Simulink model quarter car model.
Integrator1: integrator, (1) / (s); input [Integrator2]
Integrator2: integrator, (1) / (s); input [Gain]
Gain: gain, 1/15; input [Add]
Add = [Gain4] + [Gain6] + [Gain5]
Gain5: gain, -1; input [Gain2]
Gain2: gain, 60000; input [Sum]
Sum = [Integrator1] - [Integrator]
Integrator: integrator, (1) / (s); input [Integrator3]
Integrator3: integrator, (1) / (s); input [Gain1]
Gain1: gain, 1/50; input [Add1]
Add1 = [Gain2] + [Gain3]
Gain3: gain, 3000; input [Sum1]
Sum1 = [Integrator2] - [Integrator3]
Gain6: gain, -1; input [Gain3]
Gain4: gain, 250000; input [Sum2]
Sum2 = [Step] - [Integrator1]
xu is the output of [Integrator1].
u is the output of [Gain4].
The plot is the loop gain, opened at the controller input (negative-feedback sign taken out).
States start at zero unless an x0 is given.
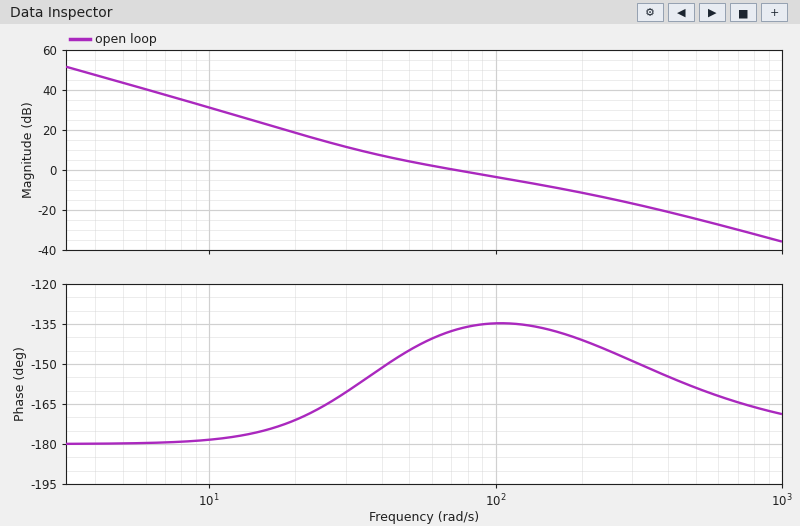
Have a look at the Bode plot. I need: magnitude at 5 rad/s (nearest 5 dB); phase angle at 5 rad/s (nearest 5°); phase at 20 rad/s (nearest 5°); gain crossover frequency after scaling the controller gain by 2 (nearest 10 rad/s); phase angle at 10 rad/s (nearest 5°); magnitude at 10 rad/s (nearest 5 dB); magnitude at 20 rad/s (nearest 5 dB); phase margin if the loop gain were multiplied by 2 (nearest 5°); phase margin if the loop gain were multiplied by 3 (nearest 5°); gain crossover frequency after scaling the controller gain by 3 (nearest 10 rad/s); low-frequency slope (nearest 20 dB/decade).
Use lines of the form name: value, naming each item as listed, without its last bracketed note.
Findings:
magnitude at 5 rad/s: 45 dB
phase angle at 5 rad/s: -180°
phase at 20 rad/s: -170°
gain crossover frequency after scaling the controller gain by 2: 130 rad/s
phase angle at 10 rad/s: -180°
magnitude at 10 rad/s: 30 dB
magnitude at 20 rad/s: 20 dB
phase margin if the loop gain were multiplied by 2: 45°
phase margin if the loop gain were multiplied by 3: 40°
gain crossover frequency after scaling the controller gain by 3: 170 rad/s
low-frequency slope: -40 dB/decade
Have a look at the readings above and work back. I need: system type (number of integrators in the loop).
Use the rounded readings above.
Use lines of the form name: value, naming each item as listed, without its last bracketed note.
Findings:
system type: 2
